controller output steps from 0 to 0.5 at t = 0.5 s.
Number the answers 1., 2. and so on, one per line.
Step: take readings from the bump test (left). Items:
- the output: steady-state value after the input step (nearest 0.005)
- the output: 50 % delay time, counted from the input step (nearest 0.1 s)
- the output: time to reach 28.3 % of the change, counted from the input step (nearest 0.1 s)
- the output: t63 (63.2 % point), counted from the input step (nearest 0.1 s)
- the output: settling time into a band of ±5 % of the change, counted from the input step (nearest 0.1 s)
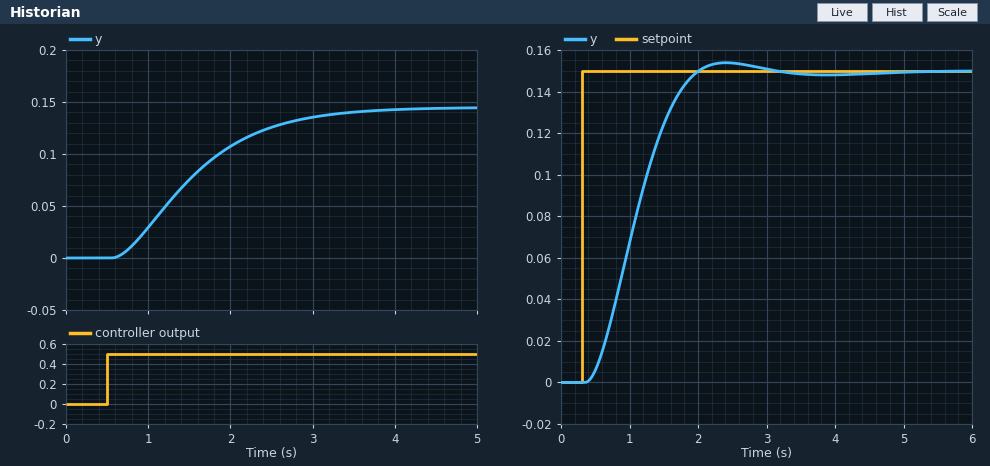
1. 0.145
2. 1.0 s
3. 0.6 s
4. 1.2 s
5. 2.7 s
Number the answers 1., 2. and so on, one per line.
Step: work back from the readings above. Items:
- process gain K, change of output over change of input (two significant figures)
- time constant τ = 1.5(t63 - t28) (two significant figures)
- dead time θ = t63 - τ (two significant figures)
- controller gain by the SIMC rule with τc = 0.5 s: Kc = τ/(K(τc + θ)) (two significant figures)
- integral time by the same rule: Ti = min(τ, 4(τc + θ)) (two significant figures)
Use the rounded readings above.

1. 0.29
2. 0.90 s
3. 0.30 s
4. 3.9
5. 0.90 s
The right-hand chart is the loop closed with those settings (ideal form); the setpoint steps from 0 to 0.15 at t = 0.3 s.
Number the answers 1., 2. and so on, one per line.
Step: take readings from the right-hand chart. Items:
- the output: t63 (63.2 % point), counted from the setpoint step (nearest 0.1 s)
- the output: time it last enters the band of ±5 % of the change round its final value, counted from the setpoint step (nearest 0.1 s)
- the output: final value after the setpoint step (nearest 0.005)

1. 0.9 s
2. 1.5 s
3. 0.150
